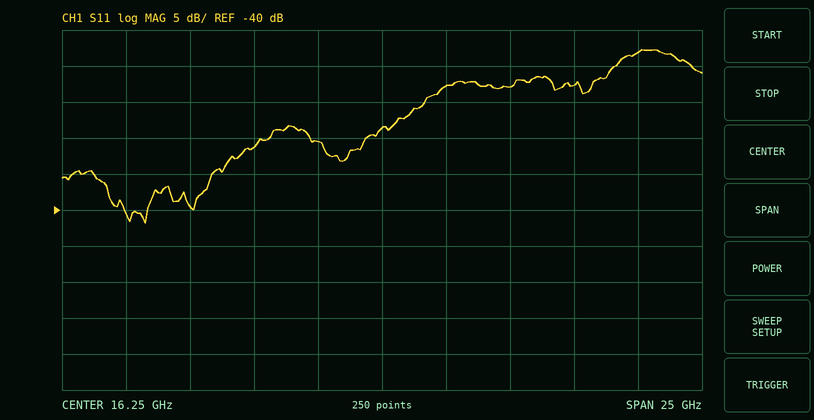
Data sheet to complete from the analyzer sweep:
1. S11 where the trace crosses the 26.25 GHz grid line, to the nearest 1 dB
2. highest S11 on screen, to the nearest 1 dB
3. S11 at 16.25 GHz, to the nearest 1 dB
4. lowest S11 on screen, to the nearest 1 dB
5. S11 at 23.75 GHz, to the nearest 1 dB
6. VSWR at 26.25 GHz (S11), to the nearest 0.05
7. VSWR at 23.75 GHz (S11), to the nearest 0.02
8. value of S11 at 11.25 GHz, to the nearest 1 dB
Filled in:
-18 dB
-18 dB
-29 dB
-42 dB
-23 dB
1.30
1.16
-31 dB
